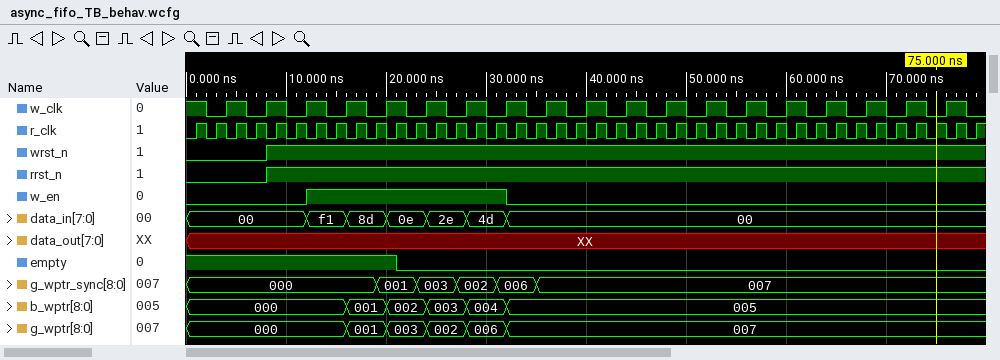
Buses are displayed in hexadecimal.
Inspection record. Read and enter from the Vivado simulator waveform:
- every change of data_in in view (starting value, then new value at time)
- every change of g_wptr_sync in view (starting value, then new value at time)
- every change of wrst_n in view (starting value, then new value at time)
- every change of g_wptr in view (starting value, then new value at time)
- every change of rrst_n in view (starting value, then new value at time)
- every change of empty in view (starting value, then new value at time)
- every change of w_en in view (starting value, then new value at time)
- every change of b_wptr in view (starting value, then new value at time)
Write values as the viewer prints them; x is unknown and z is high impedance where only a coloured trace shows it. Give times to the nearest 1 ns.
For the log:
00, f1 at 12 ns, 8d at 16 ns, 0e at 20 ns, 2e at 24 ns, 4d at 28 ns, 00 at 32 ns
000, 001 at 19 ns, 003 at 23 ns, 002 at 27 ns, 006 at 31 ns, 007 at 35 ns
0, 1 at 8 ns
000, 001 at 16 ns, 003 at 20 ns, 002 at 24 ns, 006 at 28 ns, 007 at 32 ns
0, 1 at 8 ns
1, 0 at 21 ns
0, 1 at 12 ns, 0 at 32 ns
000, 001 at 16 ns, 002 at 20 ns, 003 at 24 ns, 004 at 28 ns, 005 at 32 ns
